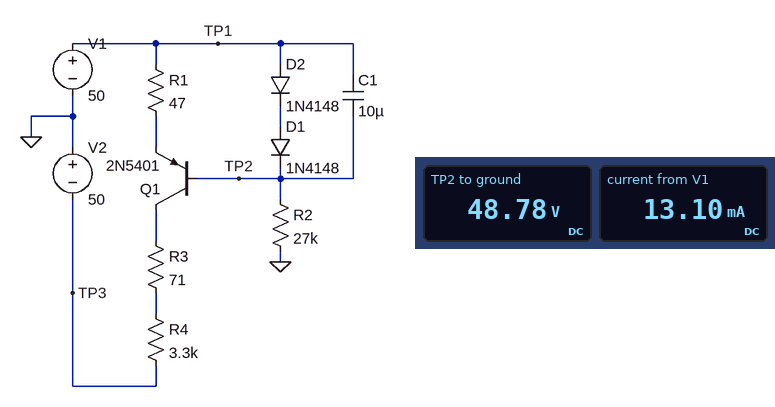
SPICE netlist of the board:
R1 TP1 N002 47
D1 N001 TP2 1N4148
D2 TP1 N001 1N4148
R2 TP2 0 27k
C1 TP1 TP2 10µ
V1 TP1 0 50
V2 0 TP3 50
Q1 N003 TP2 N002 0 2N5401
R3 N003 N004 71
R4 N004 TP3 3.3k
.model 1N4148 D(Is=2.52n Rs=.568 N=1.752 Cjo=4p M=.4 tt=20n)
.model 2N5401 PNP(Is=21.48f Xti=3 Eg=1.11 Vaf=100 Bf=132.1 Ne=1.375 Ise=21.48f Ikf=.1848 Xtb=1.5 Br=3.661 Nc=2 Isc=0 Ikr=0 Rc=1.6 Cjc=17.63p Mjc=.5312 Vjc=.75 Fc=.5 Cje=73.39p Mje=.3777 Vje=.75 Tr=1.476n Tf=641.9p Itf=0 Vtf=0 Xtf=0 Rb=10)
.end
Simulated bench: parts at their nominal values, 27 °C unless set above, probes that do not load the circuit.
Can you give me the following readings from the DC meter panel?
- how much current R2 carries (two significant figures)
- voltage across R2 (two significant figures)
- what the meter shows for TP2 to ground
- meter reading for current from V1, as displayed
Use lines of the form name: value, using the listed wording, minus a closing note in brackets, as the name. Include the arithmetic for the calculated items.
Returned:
how much current R2 carries: (48.78 V) / 27 kΩ = 1.8 mA
voltage across R2: 48.78 V = 49 V
what the meter shows for TP2 to ground: 48.78 V
meter reading for current from V1, as displayed: 13.10 mA
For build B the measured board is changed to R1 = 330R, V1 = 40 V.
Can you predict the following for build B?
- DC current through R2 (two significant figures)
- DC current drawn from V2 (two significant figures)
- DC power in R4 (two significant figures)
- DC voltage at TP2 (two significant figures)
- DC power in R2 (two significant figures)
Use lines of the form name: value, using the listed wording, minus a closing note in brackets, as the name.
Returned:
DC current through R2: 1.4 mA
DC current drawn from V2: 1.7 mA
DC power in R4: 9.7 mW
DC voltage at TP2: 39 V
DC power in R2: 56 mW
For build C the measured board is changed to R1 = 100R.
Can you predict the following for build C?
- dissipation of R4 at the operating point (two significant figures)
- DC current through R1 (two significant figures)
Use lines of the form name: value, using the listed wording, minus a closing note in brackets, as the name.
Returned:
dissipation of R4 at the operating point: 100 mW
DC current through R1: 5.6 mA
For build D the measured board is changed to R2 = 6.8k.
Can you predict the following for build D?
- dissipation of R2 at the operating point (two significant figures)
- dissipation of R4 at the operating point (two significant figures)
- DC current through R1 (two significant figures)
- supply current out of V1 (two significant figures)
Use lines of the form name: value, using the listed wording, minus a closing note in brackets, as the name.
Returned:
dissipation of R2 at the operating point: 350 mW
dissipation of R4 at the operating point: 640 mW
DC current through R1: 14 mA
supply current out of V1: 21 mA
